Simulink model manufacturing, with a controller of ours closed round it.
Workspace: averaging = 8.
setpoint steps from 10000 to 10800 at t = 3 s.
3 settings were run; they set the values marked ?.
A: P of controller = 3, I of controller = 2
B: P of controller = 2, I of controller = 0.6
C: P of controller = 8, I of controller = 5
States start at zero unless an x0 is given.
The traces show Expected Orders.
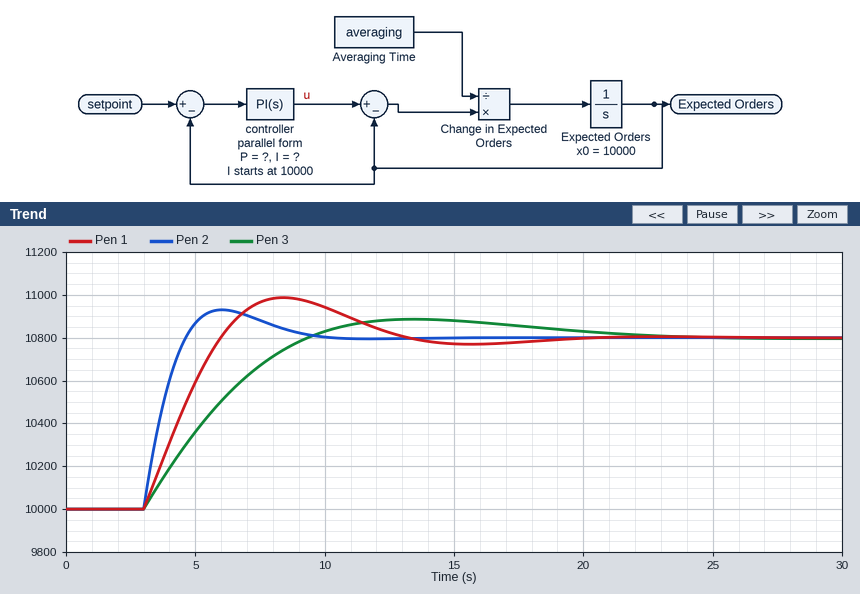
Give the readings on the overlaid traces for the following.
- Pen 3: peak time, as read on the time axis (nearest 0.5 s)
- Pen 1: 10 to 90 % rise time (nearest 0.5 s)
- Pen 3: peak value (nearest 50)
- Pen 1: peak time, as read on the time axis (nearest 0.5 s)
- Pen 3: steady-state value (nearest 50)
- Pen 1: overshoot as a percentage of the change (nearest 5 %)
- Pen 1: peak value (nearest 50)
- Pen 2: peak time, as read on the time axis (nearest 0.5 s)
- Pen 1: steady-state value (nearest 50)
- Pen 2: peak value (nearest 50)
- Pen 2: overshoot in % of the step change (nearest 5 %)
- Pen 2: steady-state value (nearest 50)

13.5 s
2.5 s
10900
8.5 s
10800
25 %
11000
6.0 s
10800
10950
15 %
10800
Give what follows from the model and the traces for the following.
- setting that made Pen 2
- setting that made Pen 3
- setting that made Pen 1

C
B
A
